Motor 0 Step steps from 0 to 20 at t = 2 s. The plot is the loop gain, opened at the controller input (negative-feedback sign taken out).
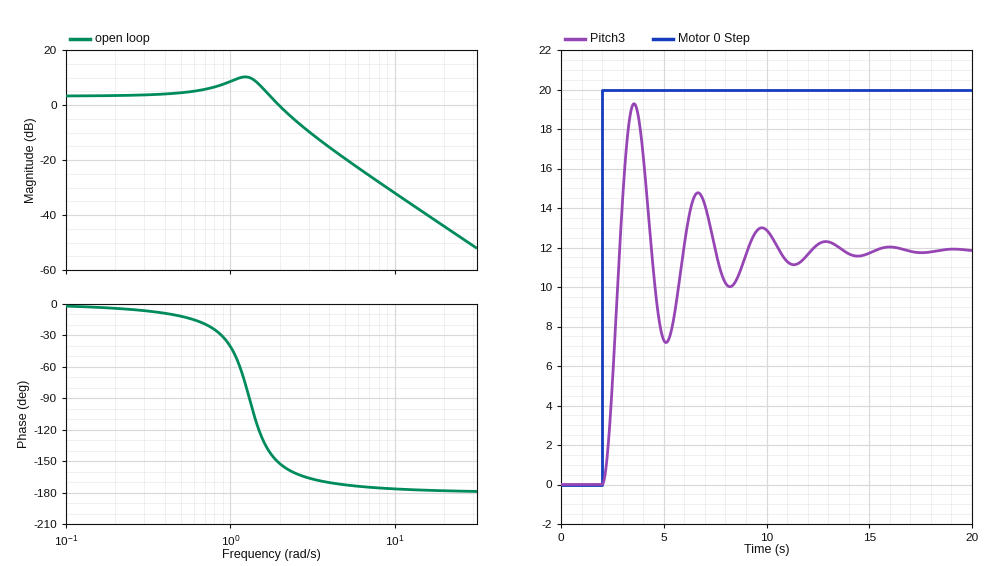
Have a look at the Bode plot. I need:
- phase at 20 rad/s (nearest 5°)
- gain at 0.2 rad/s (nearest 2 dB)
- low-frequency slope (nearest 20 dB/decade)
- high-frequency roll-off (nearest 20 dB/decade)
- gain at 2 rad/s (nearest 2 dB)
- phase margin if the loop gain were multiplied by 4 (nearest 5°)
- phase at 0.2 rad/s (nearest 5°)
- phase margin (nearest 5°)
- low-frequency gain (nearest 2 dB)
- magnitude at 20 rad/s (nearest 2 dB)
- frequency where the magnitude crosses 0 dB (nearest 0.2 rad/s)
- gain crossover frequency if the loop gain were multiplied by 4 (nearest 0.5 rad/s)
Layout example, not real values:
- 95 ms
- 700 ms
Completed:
- -180°
- 4 dB
- 0 dB/decade
- -40 dB/decade
- 0 dB
- 10°
- -5°
- 30°
- 4 dB
- -44 dB
- 2.0 rad/s
- 3.5 rad/s
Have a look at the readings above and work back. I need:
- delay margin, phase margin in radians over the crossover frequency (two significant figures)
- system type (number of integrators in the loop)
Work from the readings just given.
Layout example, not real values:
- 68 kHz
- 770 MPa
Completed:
- 0.26 s
- 0
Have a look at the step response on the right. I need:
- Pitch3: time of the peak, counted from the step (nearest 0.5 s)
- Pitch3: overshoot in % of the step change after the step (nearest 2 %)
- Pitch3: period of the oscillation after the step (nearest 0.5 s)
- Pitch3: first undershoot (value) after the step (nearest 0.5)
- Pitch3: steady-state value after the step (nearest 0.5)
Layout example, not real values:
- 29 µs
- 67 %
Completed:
- 1.5 s
- 62 %
- 3.0 s
- 7.0
- 12.0
